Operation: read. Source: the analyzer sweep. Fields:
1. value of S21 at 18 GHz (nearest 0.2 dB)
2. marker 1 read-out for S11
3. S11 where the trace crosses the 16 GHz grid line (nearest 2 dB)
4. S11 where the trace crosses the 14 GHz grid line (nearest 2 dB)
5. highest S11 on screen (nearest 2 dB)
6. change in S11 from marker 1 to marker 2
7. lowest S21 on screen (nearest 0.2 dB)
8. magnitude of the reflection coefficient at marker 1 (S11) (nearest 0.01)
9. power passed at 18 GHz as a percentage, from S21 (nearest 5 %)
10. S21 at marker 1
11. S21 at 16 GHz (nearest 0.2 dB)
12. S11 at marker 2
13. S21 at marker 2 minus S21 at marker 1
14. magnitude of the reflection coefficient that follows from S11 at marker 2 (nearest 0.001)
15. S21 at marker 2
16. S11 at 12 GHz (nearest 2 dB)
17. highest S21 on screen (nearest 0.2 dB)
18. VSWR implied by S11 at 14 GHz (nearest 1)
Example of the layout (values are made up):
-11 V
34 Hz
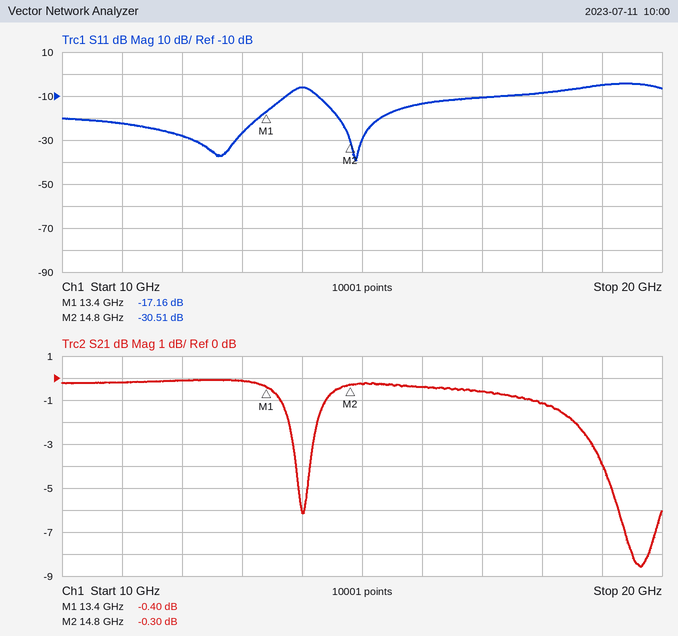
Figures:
-1.2 dB
-17.16 dB
-14 dB
-6 dB
-4 dB
-13.35 dB
-8.6 dB
0.14
75 %
-0.40 dB
-0.4 dB
-30.51 dB
0.10 dB
0.030
-0.30 dB
-28 dB
0.0 dB
3
